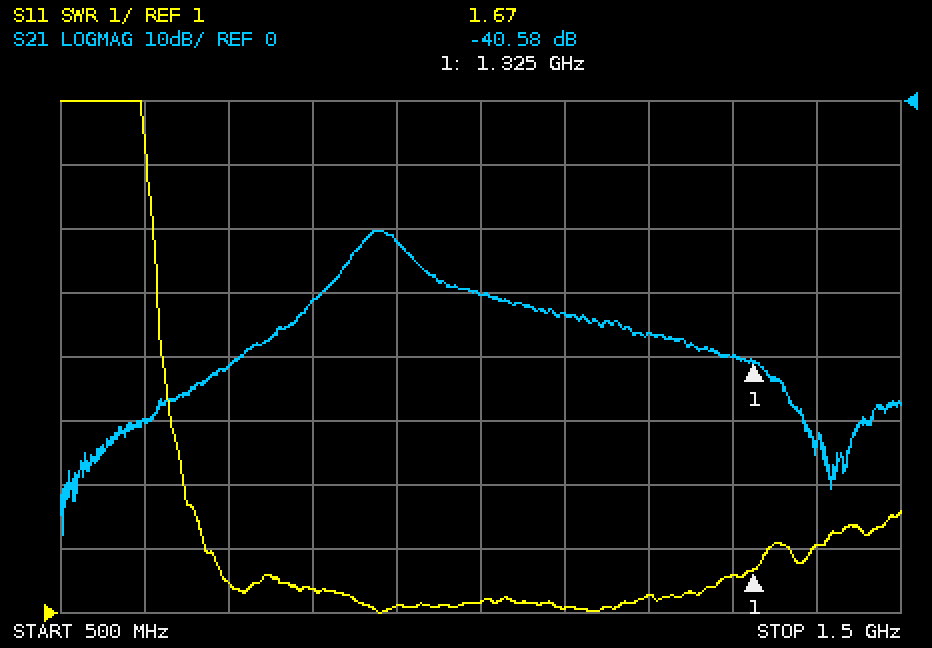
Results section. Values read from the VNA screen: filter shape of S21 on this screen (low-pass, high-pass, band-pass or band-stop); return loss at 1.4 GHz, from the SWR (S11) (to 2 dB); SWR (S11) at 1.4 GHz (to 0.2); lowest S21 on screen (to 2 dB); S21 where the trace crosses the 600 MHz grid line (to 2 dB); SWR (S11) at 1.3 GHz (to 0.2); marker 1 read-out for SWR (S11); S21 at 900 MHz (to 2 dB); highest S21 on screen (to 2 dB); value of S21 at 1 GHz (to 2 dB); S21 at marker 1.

band-pass
10 dB
2.0
-68 dB
-50 dB
1.6
1.67
-22 dB
-20 dB
-30 dB
-40.58 dB
